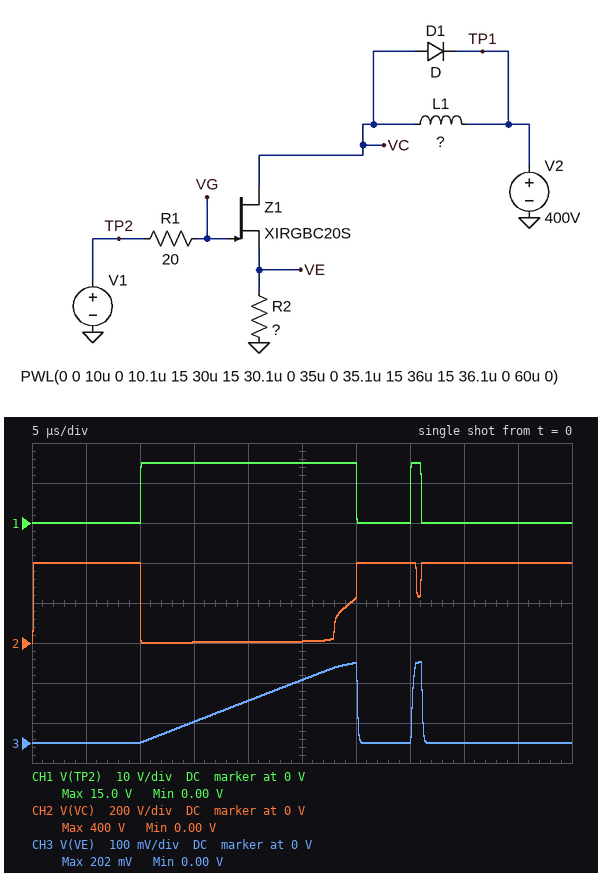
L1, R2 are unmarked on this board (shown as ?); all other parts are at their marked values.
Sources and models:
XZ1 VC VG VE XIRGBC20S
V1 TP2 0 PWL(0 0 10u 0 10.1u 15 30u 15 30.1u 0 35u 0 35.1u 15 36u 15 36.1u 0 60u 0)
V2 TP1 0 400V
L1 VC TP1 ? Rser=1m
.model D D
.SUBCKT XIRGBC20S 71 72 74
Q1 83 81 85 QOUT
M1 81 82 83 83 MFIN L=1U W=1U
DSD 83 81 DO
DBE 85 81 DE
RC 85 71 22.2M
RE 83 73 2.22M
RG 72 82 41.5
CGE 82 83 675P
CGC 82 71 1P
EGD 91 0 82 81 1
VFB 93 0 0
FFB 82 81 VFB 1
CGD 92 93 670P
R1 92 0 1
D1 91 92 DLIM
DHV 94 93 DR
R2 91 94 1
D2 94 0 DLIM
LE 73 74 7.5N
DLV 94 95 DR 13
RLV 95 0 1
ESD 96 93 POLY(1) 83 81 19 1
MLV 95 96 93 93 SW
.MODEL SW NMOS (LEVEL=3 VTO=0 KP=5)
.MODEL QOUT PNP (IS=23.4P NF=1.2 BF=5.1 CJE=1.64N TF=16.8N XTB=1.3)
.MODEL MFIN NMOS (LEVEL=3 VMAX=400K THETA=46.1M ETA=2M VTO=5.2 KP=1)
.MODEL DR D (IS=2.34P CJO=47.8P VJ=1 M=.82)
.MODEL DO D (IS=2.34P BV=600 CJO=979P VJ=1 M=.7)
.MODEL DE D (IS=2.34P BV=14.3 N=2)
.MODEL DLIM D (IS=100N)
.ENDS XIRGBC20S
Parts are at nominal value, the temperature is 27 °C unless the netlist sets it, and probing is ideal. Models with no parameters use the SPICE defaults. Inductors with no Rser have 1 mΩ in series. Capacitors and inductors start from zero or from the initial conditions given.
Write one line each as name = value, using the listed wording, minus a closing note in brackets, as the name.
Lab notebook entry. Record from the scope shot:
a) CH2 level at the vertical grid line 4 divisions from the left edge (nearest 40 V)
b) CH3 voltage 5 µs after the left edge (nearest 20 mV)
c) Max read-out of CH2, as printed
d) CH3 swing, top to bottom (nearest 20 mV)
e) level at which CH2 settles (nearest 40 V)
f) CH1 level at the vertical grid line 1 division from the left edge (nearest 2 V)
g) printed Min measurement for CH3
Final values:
CH2 level at the vertical grid line 4 divisions from the left edge = 0 V
CH3 voltage 5 µs after the left edge = 0 V
Max read-out of CH2, as printed = 400 V
CH3 swing, top to bottom = 200 mV
level at which CH2 settles = 400 V
CH1 level at the vertical grid line 1 division from the left edge = 0 V
printed Min measurement for CH3 = 0.00 V
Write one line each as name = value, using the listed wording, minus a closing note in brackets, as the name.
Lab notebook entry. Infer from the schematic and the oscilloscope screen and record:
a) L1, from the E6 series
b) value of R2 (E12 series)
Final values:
L1, from the E6 series = 68 µH
value of R2 = 1.8 mΩ
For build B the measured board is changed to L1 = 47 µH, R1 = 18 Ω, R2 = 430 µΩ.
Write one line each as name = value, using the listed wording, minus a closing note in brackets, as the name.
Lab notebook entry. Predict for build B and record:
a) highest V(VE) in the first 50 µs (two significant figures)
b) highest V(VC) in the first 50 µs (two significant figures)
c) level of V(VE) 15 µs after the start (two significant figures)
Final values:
highest V(VE) in the first 50 µs = 53 mV
highest V(VC) in the first 50 µs = 400 V
level of V(VE) 15 µs after the start = 18 mV
